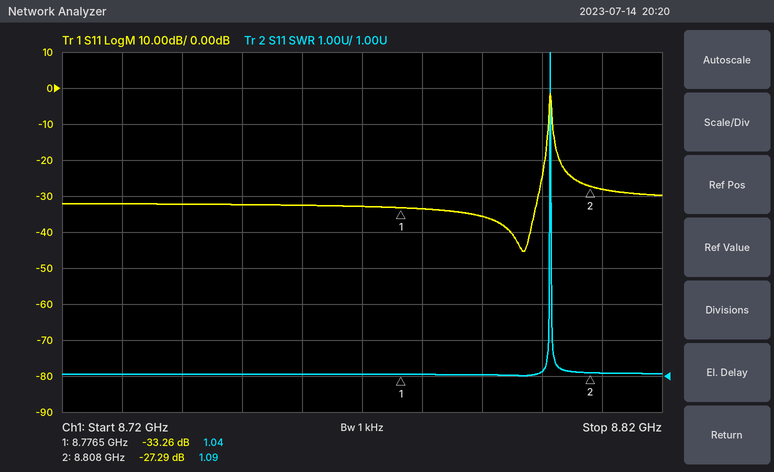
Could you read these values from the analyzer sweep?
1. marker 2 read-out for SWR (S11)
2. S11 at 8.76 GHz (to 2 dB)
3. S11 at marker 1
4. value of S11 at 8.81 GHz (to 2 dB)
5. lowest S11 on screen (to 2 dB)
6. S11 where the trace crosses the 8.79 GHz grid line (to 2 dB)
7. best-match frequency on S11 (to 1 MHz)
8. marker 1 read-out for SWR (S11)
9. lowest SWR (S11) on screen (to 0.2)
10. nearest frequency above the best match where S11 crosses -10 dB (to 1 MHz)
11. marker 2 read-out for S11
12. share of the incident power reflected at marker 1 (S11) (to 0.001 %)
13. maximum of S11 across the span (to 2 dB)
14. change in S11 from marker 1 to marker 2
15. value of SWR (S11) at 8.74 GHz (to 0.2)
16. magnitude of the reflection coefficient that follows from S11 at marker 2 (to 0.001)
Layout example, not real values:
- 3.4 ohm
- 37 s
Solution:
- 1.09
- -32 dB
- -33.26 dB
- -28 dB
- -46 dB
- -36 dB
- 8.797 GHz
- 1.04
- 1.0
- 8.801 GHz
- -27.29 dB
- 0.047 %
- -2 dB
- 5.97 dB
- 1.0
- 0.043
